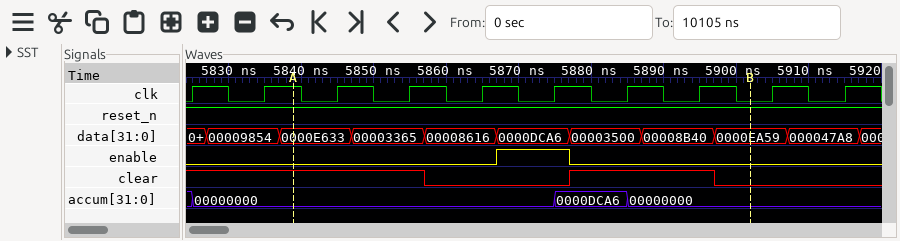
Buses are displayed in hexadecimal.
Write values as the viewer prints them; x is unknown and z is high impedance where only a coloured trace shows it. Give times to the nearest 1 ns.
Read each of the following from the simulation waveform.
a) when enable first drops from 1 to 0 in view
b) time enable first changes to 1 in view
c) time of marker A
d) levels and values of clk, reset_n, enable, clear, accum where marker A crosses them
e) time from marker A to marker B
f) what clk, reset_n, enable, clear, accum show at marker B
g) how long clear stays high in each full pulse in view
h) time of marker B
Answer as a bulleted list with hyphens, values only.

- 5877 ns
- 5867 ns
- 5839 ns
- clk=1, reset_n=1, enable=0, clear=1, accum=00000000
- 63 ns
- clk=0, reset_n=1, enable=0, clear=0, accum=00000000
- 20 ns
- 5902 ns
